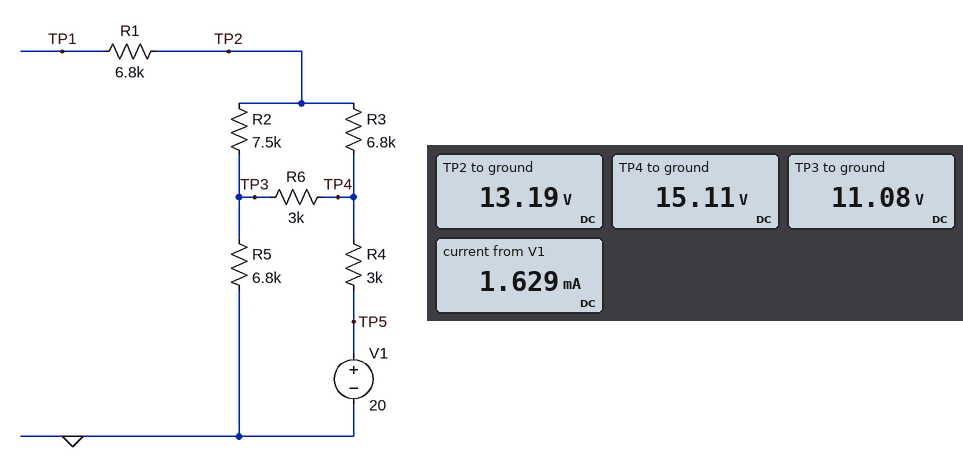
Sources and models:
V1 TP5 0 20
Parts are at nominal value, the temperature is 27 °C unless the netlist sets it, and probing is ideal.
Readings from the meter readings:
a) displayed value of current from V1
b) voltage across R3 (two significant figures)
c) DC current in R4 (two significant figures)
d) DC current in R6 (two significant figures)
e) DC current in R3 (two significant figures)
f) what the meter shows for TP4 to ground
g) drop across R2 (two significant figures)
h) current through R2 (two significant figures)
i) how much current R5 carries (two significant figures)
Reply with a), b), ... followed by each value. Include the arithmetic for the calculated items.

a) 1.629 mA
b) 15.11 V - 13.19 V = 1.9 V
c) (20 V - 15.11 V) / 3 kΩ = 1.6 mA
d) (15.11 V - 11.08 V) / 3 kΩ = 1.3 mA
e) (15.11 V - 13.19 V) / 6.8 kΩ = 280 µA
f) 15.11 V
g) 13.19 V - 11.08 V = 2.1 V
h) (13.19 V - 11.08 V) / 7.5 kΩ = 280 µA
i) (11.08 V) / 6.8 kΩ = 1.6 mA
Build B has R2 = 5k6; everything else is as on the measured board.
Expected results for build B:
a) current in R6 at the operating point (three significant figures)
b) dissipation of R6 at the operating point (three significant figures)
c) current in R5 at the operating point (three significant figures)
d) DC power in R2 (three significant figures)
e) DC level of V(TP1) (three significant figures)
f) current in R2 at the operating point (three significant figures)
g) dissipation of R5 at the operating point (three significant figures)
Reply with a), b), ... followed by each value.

a) 1.32 mA
b) 5.21 mW
c) 1.64 mA
d) 570 µW
e) 12.9 V
f) 319 µA
g) 18.2 mW
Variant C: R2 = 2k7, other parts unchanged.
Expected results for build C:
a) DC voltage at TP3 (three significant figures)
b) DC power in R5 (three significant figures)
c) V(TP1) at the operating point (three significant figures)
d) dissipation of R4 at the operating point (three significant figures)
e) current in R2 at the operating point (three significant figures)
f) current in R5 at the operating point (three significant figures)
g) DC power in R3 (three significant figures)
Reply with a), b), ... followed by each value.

a) 11.3 V
b) 18.6 mW
c) 12.3 V
d) 8.22 mW
e) 397 µA
f) 1.66 mA
g) 1.07 mW
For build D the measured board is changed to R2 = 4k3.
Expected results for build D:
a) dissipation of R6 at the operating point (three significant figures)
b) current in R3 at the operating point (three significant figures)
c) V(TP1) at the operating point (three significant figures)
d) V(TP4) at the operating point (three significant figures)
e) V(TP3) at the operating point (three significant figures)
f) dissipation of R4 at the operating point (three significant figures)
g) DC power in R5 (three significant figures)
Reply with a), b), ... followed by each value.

a) 5.03 mW
b) 350 µA
c) 12.7 V
d) 15.1 V
e) 11.2 V
f) 8.11 mW
g) 18.4 mW
